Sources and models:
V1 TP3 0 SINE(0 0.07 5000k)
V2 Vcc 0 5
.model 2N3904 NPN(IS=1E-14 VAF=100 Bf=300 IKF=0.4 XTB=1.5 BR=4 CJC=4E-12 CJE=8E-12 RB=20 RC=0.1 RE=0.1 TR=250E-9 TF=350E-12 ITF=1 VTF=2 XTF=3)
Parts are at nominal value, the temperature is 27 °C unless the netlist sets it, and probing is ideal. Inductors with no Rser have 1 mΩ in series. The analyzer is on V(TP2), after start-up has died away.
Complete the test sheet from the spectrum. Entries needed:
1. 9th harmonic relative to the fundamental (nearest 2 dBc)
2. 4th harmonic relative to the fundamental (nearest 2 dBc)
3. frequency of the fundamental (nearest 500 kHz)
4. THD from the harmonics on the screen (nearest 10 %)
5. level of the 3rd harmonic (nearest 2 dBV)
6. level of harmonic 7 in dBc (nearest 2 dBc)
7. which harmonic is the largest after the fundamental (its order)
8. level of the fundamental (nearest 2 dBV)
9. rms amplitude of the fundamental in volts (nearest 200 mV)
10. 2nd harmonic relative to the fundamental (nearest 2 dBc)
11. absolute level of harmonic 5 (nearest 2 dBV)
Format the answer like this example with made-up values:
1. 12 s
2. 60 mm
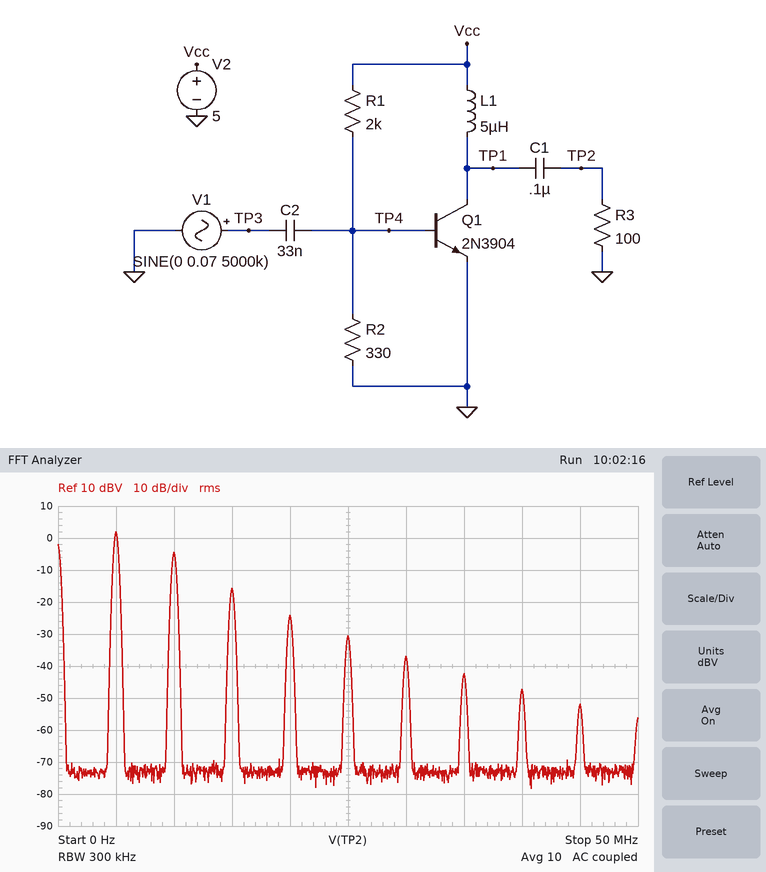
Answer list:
1. -54 dBc
2. -26 dBc
3. 5.0 MHz
4. 50 %
5. -16 dBV
6. -44 dBc
7. 2
8. 2 dBV
9. 1.2 V
10. -6 dBc
11. -30 dBV
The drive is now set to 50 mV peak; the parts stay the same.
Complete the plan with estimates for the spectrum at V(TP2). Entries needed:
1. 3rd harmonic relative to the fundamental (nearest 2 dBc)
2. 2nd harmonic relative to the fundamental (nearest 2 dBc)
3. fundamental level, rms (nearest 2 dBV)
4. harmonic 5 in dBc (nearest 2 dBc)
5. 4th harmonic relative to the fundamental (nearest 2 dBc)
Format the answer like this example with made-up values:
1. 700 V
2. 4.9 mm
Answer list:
1. -20 dBc
2. -8 dBc
3. -2 dBV
4. -40 dBc
5. -32 dBc
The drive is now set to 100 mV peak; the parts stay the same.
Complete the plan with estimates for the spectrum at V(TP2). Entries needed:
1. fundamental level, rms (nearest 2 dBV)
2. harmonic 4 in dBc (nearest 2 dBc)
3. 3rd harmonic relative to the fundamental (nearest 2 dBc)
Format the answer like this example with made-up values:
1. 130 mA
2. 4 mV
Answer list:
1. 6 dBV
2. -22 dBc
3. -16 dBc
